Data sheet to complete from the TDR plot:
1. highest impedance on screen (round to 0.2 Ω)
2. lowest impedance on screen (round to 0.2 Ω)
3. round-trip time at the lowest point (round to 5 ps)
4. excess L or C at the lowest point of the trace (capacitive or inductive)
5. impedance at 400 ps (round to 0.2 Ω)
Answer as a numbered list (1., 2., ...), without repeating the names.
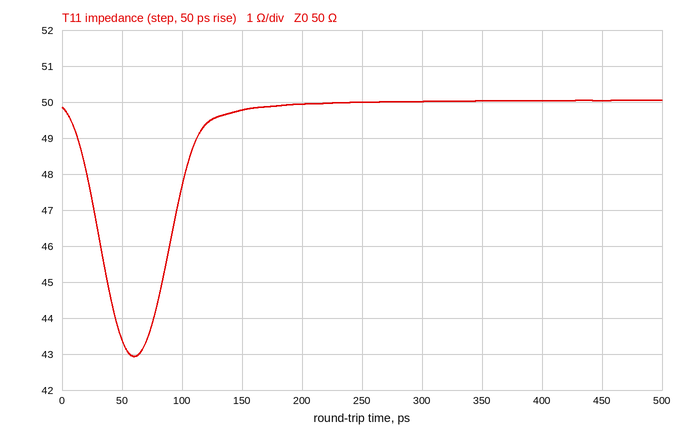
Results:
1. 50.0 Ω
2. 43.0 Ω
3. 60 ps
4. capacitive
5. 50.0 Ω
